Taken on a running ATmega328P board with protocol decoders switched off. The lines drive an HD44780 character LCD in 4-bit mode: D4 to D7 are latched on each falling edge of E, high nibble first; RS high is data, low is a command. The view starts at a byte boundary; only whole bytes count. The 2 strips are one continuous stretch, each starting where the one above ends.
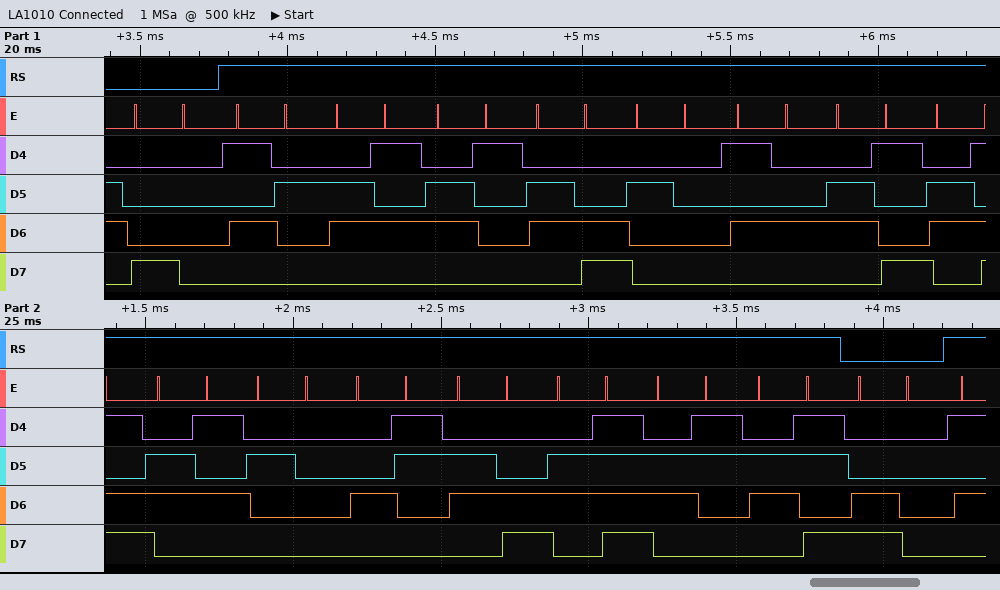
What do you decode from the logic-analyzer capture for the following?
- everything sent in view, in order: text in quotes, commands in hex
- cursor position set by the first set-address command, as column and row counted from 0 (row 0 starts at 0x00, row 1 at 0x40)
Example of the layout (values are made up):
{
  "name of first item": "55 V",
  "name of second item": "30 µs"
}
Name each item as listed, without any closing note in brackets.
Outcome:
{
  "everything sent in view, in order: text in quotes, commands in hex": "0x80 \"Real Time Clock\" 0xC0",
  "cursor position set by the first set-address command, as column and row counted from 0": "column 0, row 0"
}
